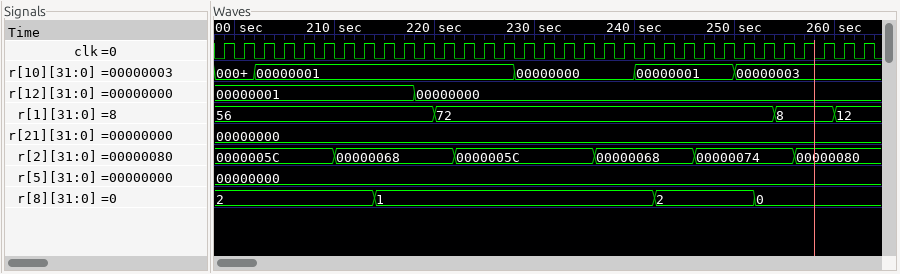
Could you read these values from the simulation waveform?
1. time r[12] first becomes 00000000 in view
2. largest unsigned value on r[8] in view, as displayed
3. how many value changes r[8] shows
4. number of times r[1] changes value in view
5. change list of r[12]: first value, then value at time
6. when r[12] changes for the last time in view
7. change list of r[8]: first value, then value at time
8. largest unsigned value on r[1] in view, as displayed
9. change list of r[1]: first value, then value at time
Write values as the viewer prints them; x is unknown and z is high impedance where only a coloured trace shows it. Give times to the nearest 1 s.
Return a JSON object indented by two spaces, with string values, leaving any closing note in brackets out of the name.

{
  "time r[12] first becomes 00000000 in view": "218 s",
  "largest unsigned value on r[8] in view, as displayed": "2",
  "how many value changes r[8] shows": "3",
  "number of times r[1] changes value in view": "3",
  "change list of r[12]: first value, then value at time": "00000001, 00000000 at 218 s",
  "when r[12] changes for the last time in view": "218 s",
  "change list of r[8]: first value, then value at time": "2, 1 at 214 s, 2 at 242 s, 0 at 252 s",
  "largest unsigned value on r[1] in view, as displayed": "72",
  "change list of r[1]: first value, then value at time": "56, 72 at 220 s, 8 at 254 s, 12 at 260 s"
}
